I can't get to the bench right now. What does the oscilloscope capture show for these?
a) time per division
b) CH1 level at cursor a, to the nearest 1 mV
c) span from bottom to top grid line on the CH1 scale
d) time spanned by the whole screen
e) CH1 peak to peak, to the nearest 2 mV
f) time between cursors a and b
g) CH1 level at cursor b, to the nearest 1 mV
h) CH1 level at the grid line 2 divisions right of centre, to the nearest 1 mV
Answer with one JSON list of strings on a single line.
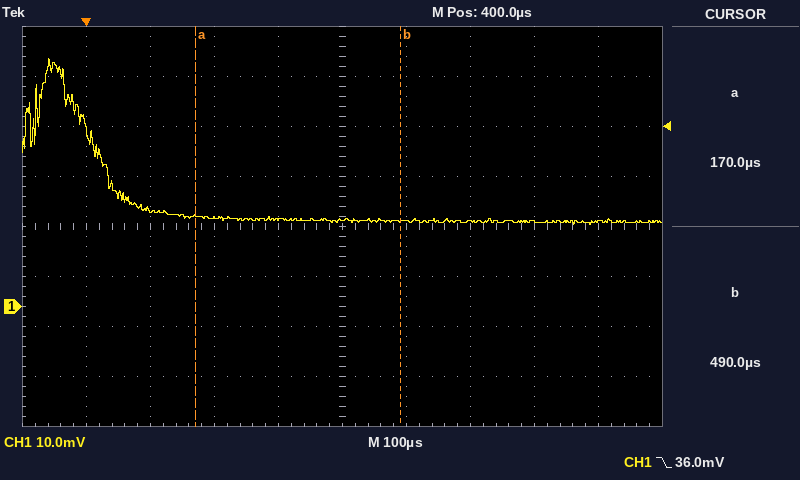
["100 µs", "18 mV", "80 mV", "1 ms", "34 mV", "320 µs", "17 mV", "17 mV"]
